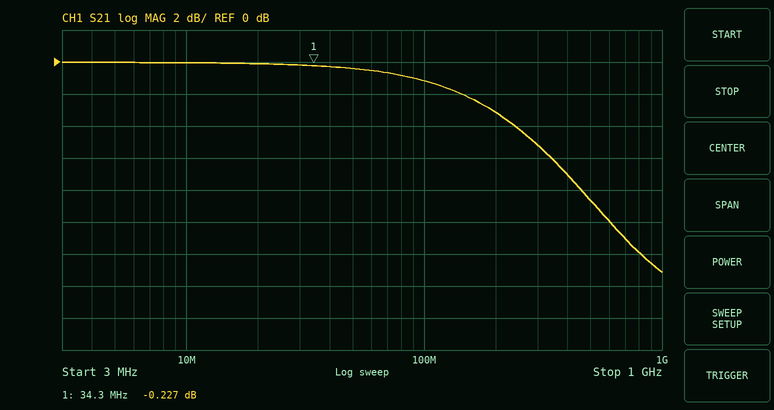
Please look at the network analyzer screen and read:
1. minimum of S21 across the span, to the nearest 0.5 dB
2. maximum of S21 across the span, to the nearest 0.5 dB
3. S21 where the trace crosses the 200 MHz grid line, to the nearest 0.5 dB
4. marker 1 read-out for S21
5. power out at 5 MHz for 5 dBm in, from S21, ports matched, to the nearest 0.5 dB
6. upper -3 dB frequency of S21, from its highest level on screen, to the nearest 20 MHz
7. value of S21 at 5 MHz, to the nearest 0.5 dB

-13.0 dB
0.0 dB
-3.0 dB
-0.227 dB
5.0 dBm
200 MHz
0.0 dB
